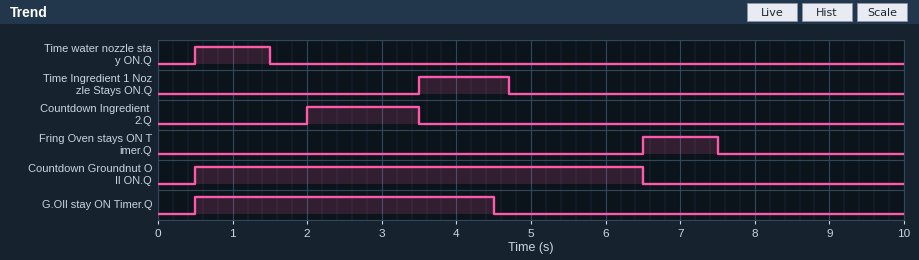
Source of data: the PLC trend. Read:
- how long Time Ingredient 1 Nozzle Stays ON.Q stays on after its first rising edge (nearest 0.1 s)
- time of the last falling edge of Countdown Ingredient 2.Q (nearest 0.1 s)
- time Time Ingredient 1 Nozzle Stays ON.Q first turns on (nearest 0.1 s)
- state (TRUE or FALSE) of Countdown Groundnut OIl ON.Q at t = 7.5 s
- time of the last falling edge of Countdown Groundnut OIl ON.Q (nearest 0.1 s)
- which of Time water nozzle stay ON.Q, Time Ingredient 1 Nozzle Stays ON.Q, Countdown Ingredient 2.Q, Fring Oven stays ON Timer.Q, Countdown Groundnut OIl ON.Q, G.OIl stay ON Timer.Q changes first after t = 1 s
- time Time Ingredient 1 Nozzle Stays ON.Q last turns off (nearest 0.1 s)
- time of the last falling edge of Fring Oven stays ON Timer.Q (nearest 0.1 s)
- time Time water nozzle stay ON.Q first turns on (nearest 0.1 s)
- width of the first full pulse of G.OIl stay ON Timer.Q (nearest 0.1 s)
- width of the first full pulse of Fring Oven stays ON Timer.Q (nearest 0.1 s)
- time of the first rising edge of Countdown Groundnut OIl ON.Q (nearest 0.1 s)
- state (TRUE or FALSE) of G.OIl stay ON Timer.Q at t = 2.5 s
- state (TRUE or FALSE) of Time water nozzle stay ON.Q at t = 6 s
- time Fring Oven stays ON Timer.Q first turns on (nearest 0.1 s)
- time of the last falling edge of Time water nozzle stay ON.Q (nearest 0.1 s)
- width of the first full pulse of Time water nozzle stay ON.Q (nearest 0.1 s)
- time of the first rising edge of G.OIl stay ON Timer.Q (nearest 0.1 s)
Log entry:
1.2 s
3.5 s
3.5 s
FALSE
6.5 s
Time water nozzle stay ON.Q
4.7 s
7.5 s
0.5 s
4.0 s
1.0 s
0.5 s
TRUE
FALSE
6.5 s
1.5 s
1.0 s
0.5 s
